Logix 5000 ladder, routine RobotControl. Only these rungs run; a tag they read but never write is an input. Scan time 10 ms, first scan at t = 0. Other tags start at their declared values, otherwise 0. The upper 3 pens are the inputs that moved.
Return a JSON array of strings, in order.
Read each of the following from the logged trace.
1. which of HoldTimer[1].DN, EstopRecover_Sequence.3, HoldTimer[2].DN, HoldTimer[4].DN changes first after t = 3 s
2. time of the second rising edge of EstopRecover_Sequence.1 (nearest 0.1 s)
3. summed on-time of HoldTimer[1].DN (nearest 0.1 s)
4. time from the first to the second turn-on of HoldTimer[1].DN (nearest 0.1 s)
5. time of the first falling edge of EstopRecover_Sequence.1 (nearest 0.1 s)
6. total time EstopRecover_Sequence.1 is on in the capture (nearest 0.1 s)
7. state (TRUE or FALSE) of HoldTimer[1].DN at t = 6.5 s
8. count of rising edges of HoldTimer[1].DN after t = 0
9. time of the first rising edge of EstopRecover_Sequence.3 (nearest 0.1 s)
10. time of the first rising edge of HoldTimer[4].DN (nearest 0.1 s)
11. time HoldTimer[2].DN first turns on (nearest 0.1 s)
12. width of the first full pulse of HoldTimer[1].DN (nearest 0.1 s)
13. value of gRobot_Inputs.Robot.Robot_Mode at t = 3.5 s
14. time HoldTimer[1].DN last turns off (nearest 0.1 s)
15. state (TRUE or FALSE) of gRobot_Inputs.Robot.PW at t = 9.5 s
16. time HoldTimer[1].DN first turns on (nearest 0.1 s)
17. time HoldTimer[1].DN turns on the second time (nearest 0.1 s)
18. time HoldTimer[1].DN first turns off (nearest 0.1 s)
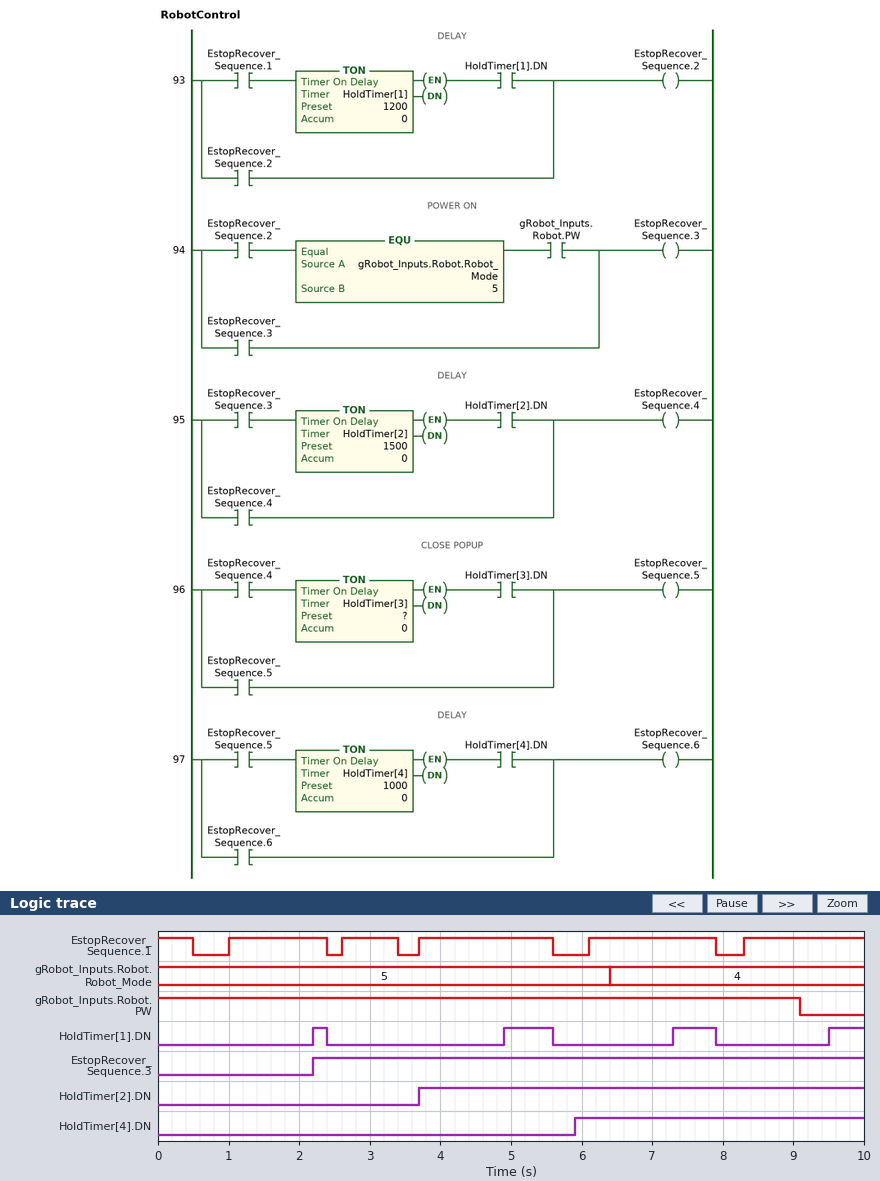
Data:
["HoldTimer[2].DN", "2.6 s", "2.0 s", "2.7 s", "0.5 s", "8.1 s", "FALSE", "4", "2.2 s", "5.9 s", "3.7 s", "0.2 s", "5", "7.9 s", "FALSE", "2.2 s", "4.9 s", "2.4 s"]
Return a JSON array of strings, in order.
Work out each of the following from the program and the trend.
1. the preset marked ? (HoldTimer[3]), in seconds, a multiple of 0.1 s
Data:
["1.2 s"]
